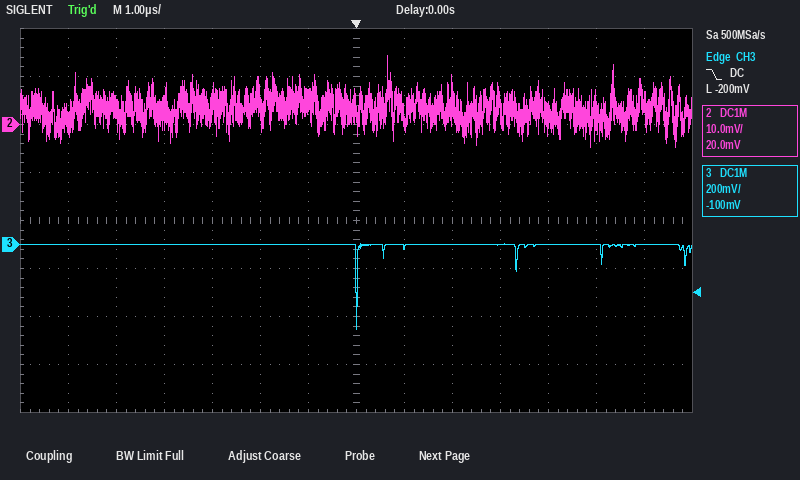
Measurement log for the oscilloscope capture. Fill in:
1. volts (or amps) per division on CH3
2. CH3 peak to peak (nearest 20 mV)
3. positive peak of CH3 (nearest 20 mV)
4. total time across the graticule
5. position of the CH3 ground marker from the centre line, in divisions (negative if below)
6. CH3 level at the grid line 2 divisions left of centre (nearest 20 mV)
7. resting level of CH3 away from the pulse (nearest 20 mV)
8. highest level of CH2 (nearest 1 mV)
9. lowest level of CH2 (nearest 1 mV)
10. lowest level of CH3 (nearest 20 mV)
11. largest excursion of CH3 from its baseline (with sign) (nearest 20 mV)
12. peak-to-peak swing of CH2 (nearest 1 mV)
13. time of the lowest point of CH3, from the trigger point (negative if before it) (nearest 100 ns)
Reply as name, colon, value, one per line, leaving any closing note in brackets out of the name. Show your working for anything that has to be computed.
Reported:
volts (or amps) per division on CH3: 200 mV
CH3 peak to peak: 0 mV − (-360 mV) = 360 mV
positive peak of CH3: 0 mV
total time across the graticule: 14 µs
position of the CH3 ground marker from the centre line, in divisions: -0.5 div
CH3 level at the grid line 2 divisions left of centre: 0 mV
resting level of CH3 away from the pulse: 0 mV
highest level of CH2: 14 mV
lowest level of CH2: -5 mV
lowest level of CH3: -360 mV
largest excursion of CH3 from its baseline (with sign): -360 mV − (0 mV) = -360 mV
peak-to-peak swing of CH2: 14 mV − (-5 mV) = 19 mV
time of the lowest point of CH3, from the trigger point (negative if before it): 0.0 µs
